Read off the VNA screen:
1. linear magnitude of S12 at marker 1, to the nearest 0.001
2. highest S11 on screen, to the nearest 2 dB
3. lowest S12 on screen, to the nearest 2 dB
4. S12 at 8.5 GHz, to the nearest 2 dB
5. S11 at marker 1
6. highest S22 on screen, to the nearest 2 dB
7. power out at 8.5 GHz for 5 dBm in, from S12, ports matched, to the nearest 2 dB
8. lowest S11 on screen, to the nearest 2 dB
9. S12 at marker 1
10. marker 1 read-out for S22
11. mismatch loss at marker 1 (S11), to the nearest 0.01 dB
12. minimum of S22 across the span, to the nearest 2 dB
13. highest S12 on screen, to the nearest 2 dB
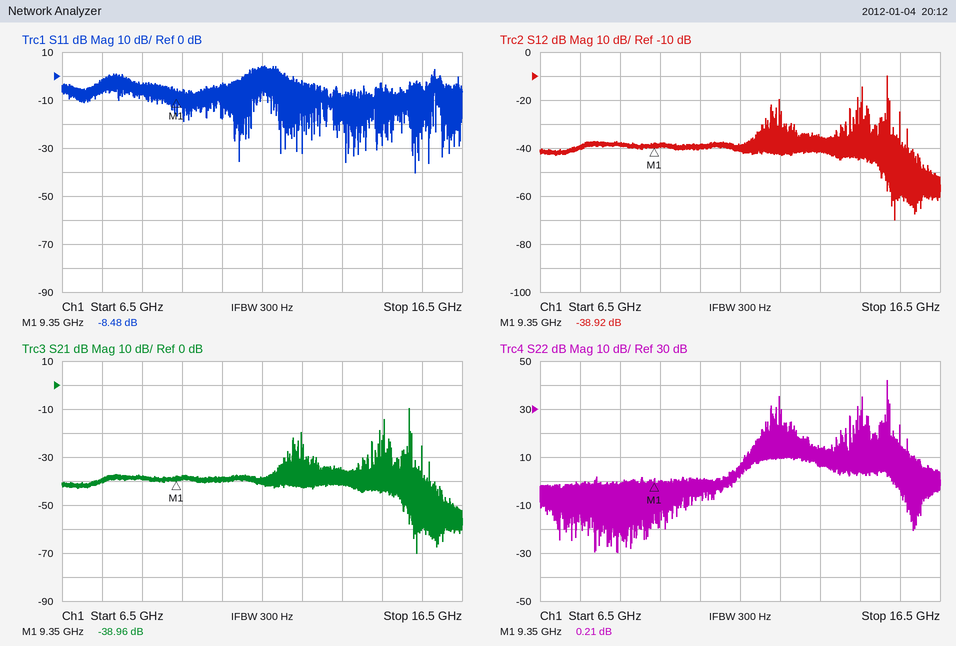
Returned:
0.011
4 dB
-70 dB
-38 dB
-8.48 dB
42 dB
-34 dBm
-40 dB
-38.92 dB
0.21 dB
0.66 dB
-30 dB
-10 dB
